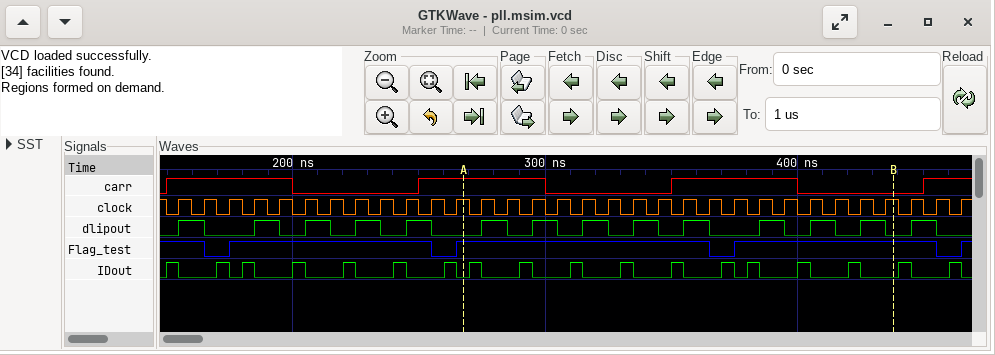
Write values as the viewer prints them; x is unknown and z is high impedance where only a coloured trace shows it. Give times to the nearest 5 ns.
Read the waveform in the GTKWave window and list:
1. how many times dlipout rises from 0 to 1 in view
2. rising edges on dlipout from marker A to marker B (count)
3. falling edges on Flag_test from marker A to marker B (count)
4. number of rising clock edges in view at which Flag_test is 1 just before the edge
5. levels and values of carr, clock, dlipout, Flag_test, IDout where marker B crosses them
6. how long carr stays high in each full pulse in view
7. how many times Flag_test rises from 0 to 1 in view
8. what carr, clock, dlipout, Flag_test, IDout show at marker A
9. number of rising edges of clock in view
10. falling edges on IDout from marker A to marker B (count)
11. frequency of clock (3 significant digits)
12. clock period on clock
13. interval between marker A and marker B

14
8
1
28
carr=0, clock=1, dlipout=0, Flag_test=1, IDout=0
50 ns, 50 ns, 50 ns
4
carr=1, clock=1, dlipout=0, Flag_test=1, IDout=0
32
9
100 MHz
10 ns
170 ns
